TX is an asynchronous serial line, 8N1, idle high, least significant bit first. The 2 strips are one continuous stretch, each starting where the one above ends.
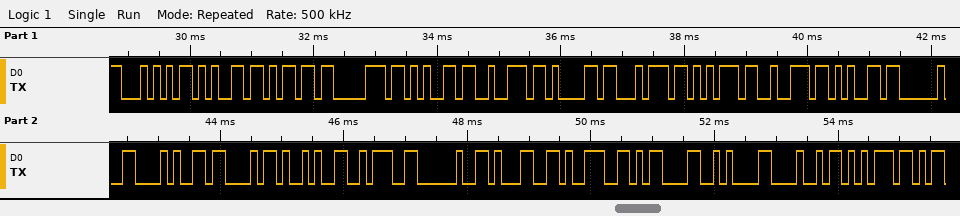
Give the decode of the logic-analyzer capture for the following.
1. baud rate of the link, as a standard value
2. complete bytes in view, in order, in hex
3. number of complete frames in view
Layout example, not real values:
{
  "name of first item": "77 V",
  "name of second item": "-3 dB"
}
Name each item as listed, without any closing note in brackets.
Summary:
{
  "baud rate of the link, as a standard value": "9600 baud",
  "complete bytes in view, in order, in hex": "54 65 6D 70 65 72 61 74 75 72 65 20 28 43 29 3A 20 31 39 0D 0A 48 75",
  "number of complete frames in view": "23"
}
